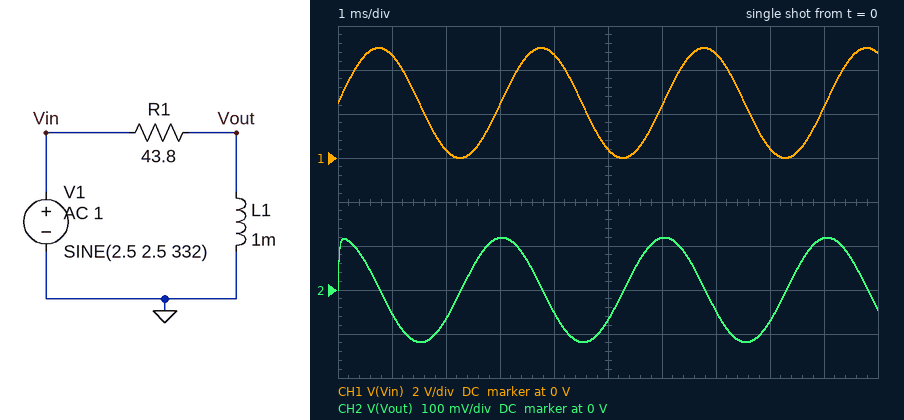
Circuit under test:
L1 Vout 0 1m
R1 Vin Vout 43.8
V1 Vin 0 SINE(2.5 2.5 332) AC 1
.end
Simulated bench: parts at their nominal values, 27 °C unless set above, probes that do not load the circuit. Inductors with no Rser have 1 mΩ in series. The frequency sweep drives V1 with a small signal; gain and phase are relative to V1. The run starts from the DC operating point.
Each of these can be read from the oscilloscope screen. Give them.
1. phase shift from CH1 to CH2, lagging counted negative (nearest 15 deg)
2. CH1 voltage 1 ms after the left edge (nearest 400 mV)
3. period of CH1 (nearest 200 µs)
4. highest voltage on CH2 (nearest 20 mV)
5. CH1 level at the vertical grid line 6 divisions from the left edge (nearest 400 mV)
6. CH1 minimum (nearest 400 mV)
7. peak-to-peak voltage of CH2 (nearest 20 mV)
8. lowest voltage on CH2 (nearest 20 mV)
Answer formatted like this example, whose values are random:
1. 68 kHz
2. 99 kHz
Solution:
1. 90 deg
2. 4.8 V
3. 3.0 ms
4. 120 mV
5. 2.4 V
6. 0 V
7. 240 mV
8. -120 mV
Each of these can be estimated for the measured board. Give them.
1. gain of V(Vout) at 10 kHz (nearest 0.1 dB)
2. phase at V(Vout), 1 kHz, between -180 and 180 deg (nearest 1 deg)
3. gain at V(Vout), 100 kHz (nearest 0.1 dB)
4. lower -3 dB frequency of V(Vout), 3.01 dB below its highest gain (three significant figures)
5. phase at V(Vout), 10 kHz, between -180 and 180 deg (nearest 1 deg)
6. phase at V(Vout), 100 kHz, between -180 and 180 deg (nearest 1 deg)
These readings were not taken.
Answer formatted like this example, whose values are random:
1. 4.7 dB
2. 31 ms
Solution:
1. -1.7 dB
2. 82 deg
3. 0 dB
4. 6.97 kHz
5. 35 deg
6. 4 deg
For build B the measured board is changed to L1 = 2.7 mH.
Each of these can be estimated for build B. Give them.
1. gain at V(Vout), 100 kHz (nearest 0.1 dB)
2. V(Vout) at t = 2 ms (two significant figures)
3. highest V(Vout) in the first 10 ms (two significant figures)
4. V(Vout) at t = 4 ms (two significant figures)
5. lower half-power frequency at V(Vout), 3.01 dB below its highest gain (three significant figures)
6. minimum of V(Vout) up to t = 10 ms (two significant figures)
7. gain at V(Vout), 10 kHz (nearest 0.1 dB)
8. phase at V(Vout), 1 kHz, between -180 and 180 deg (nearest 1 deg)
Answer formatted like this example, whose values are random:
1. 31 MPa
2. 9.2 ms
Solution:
1. 0 dB
2. -200 mV
3. 320 mV
4. -110 mV
5. 2.58 kHz
6. -320 mV
7. -0.3 dB
8. 69 deg
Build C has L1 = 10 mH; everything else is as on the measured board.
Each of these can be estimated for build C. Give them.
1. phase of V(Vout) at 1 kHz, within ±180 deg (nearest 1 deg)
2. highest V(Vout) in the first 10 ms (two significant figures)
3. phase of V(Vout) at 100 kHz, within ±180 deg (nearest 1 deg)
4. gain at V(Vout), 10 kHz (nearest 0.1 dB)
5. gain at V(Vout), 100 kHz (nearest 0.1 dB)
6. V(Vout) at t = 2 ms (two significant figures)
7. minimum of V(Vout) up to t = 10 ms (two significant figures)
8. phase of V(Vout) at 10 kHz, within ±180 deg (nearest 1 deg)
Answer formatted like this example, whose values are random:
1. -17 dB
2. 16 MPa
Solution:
1. 35 deg
2. 1.1 V
3. 0 deg
4. 0 dB
5. 0 dB
6. -900 mV
7. -1.1 V
8. 4 deg
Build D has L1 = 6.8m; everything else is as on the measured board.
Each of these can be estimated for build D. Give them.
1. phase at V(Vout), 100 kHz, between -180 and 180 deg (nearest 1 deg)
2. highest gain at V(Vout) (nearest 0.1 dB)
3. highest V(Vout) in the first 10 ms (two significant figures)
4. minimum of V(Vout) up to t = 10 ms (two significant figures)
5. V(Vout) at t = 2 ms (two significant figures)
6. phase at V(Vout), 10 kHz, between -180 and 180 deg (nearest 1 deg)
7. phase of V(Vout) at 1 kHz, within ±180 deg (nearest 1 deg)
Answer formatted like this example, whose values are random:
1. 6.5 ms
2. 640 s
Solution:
1. 1 deg
2. 0 dB
3. 770 mV
4. -770 mV
5. -580 mV
6. 6 deg
7. 46 deg
